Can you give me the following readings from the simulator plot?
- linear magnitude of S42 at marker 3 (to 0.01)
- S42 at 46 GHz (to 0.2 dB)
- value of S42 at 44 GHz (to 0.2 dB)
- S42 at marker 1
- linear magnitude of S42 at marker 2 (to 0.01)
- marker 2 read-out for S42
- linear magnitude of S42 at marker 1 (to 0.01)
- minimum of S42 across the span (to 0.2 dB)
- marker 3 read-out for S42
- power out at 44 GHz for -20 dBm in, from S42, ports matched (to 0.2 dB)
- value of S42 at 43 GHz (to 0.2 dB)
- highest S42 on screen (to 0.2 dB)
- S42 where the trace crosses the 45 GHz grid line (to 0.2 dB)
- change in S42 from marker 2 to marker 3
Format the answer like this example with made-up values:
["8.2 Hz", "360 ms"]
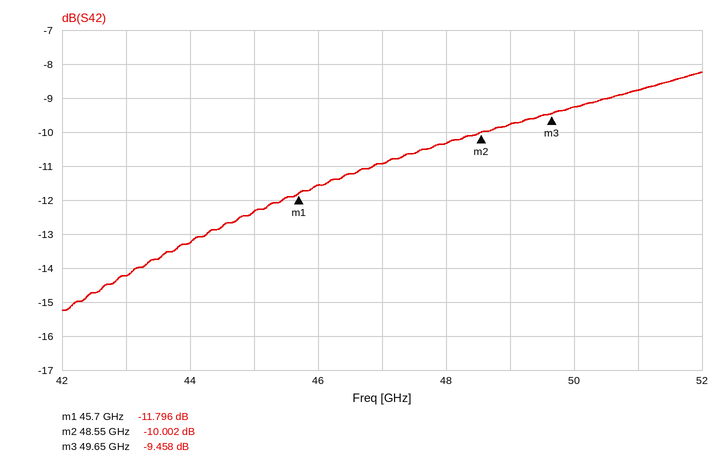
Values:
["0.34", "-11.6 dB", "-13.2 dB", "-11.796 dB", "0.32", "-10.002 dB", "0.26", "-15.2 dB", "-9.458 dB", "-33.2 dBm", "-14.2 dB", "-8.2 dB", "-12.4 dB", "0.544 dB"]
